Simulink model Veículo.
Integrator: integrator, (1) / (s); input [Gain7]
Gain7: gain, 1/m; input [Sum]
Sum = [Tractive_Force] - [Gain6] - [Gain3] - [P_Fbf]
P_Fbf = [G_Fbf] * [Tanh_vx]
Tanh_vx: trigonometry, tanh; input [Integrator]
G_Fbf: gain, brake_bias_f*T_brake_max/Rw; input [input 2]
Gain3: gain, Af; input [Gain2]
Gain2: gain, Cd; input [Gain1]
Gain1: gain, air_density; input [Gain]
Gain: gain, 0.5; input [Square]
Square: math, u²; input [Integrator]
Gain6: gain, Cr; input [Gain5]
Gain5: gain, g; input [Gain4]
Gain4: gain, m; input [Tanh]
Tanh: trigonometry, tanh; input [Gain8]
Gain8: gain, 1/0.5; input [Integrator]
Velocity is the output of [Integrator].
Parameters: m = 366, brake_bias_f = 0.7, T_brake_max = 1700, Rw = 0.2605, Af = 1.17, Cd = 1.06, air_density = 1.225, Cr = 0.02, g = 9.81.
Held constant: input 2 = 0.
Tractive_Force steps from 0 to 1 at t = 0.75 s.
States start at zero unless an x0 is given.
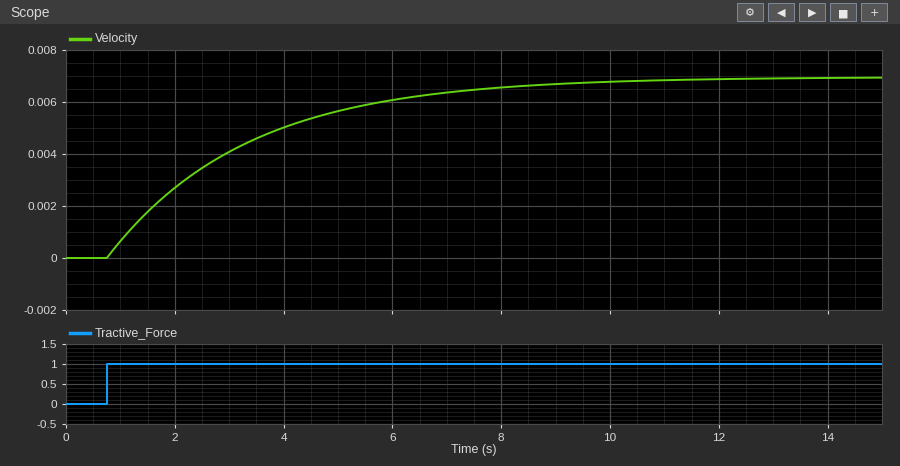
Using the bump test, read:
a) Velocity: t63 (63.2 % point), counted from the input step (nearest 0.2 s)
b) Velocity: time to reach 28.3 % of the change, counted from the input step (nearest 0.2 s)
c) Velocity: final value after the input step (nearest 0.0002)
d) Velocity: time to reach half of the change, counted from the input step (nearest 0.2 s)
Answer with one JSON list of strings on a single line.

["2.6 s", "0.8 s", "0.0070", "1.8 s"]
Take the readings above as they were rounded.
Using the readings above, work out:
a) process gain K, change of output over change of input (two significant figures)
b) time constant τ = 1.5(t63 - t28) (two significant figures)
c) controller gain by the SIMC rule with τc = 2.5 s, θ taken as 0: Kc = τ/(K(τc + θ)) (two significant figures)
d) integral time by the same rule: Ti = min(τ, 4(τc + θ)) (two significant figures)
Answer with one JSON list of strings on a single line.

["0.0070", "2.7 s", "150", "2.7 s"]
